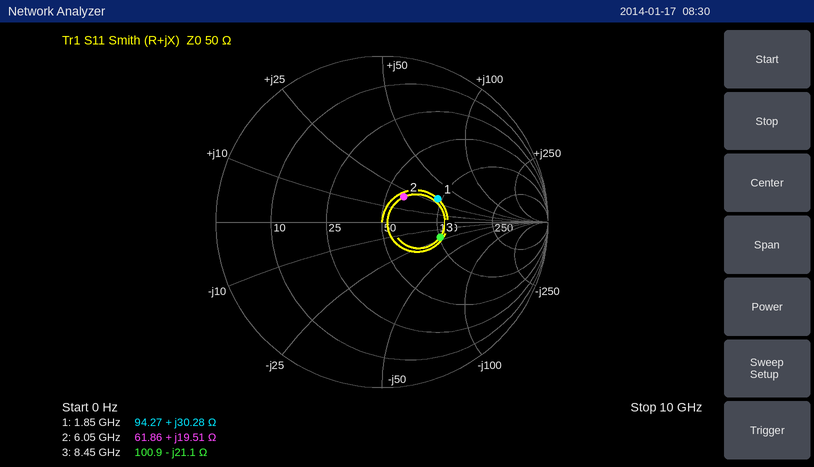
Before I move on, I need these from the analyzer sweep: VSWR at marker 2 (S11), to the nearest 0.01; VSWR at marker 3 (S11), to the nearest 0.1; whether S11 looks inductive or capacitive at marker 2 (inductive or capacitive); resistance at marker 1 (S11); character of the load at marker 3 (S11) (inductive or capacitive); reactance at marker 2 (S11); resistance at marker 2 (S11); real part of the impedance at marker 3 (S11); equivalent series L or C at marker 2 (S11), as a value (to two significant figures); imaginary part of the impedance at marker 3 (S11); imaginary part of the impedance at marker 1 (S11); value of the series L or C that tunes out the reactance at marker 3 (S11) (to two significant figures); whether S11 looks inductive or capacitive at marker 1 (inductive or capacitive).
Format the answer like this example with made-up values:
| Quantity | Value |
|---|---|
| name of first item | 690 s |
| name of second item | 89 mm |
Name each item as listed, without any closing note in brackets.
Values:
| Quantity | Value |
|---|---|
| VSWR at marker 2 (S11), to the nearest 0.01 | 1.50 |
| VSWR at marker 3 (S11), to the nearest 0.1 | 2.1 |
| whether S11 looks inductive or capacitive at marker 2 | inductive |
| resistance at marker 1 | 94.27 Ω |
| character of the load at marker 3 (S11) | capacitive |
| reactance at marker 2 | +19.51 Ω |
| resistance at marker 2 | 61.86 Ω |
| real part of the impedance at marker 3 | 100.9 Ω |
| equivalent series L or C at marker 2 (S11), as a value | 510 pH |
| imaginary part of the impedance at marker 3 | -21.1 Ω |
| imaginary part of the impedance at marker 1 | +30.28 Ω |
| value of the series L or C that tunes out the reactance at marker 3 (S11) | 400 pH |
| whether S11 looks inductive or capacitive at marker 1 | inductive |
